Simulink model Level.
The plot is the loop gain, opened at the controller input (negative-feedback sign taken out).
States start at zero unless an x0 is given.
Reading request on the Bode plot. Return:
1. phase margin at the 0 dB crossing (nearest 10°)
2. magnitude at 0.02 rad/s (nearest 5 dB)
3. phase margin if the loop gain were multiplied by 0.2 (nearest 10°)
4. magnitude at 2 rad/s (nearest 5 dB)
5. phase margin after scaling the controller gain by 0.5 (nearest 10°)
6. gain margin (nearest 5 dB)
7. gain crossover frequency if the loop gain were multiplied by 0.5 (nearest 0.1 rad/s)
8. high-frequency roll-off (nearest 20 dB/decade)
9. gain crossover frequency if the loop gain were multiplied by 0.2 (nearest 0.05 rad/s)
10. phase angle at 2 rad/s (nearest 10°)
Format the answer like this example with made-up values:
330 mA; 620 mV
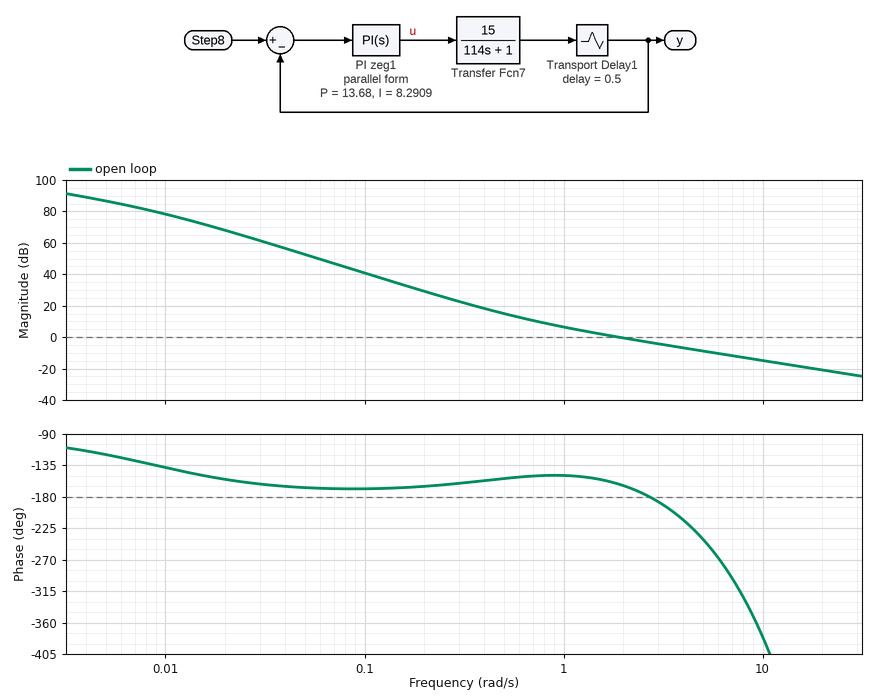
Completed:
20°; 70 dB; 30°; 0 dB; 30°; 5 dB; 1.0 rad/s; -20 dB/decade; 0.55 rad/s; -160°
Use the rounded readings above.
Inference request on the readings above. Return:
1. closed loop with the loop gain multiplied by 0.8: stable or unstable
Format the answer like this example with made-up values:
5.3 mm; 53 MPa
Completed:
stable
